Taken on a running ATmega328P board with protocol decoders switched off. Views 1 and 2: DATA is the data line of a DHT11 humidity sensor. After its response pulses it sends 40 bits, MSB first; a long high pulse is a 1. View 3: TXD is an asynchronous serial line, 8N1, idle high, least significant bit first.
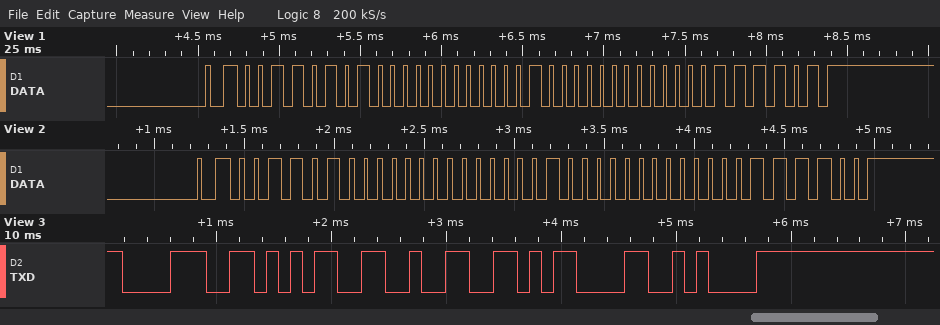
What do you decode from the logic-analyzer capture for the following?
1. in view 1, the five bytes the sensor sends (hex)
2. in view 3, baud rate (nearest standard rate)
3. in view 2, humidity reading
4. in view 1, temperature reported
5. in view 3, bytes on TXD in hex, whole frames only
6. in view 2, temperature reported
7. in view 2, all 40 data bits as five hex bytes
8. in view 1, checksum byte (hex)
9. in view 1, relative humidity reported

35 00 08 00 3D
9600 baud
52 %
8.0 °C
0x38 0x35 0x32 0x0D 0x0A
8.0 °C
34 00 08 00 3C
0x3D
53 %
